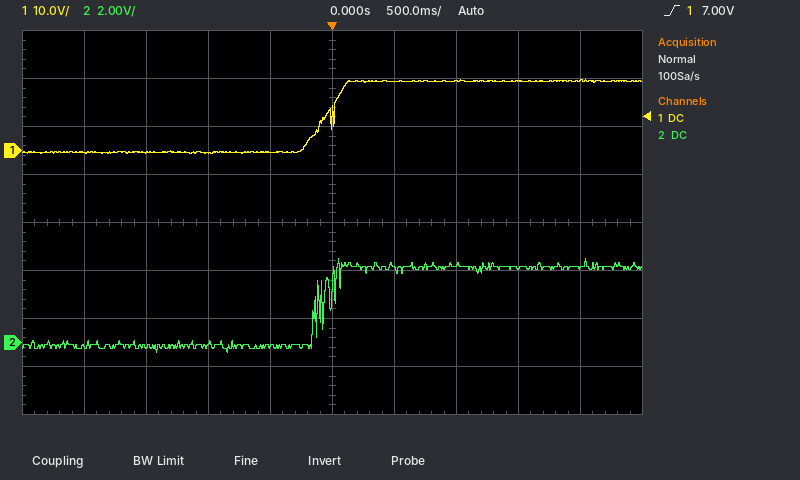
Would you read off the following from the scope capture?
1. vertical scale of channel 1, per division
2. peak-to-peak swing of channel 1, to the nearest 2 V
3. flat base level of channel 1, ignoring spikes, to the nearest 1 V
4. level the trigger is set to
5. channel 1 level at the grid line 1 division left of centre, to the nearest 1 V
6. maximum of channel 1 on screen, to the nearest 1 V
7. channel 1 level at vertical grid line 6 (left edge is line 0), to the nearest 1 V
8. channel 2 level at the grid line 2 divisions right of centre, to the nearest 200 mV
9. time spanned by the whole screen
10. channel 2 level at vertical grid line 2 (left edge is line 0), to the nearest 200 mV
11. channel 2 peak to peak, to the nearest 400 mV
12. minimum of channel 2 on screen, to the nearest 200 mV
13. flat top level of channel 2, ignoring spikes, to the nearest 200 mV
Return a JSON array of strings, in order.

["10 V", "16 V", "0 V", "7.00 V", "0 V", "15 V", "14 V", "3.2 V", "5 s", "-200 mV", "4.0 V", "-400 mV", "3.2 V"]
